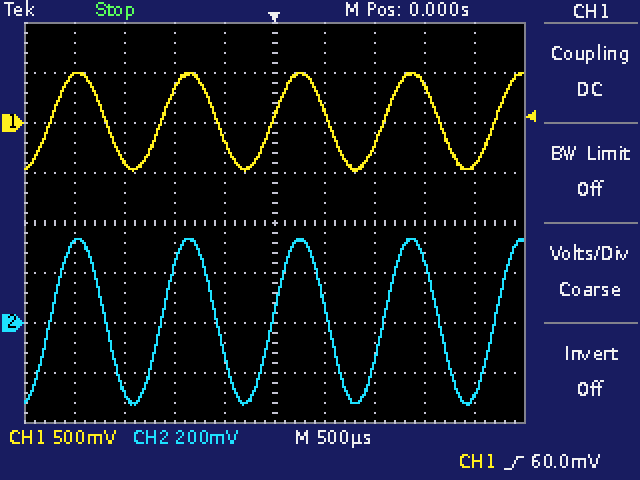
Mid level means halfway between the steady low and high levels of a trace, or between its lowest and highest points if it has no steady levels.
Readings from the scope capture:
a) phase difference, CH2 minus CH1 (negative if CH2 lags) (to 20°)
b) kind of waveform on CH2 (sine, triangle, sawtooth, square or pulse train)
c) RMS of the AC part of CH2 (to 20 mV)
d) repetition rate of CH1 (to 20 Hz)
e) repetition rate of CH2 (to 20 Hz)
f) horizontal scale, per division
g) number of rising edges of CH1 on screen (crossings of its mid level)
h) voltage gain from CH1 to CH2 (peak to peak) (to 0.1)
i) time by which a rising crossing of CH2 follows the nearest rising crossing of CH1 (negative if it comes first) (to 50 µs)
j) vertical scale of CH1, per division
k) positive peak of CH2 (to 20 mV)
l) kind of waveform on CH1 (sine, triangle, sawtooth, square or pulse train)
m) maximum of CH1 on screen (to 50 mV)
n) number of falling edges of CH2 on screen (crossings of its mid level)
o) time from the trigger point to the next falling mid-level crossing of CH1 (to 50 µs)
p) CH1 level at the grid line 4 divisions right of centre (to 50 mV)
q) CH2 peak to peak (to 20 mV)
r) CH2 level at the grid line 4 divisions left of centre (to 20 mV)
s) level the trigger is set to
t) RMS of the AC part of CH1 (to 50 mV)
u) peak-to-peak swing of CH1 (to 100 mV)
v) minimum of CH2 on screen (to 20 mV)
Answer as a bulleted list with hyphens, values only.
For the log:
- 0°
- sine
- 240 mV
- 900 Hz
- 900 Hz
- 500 µs
- 5
- 0.7
- 0 µs
- 500 mV
- 340 mV
- sine
- 500 mV
- 4
- 550 µs
- -400 mV
- 660 mV
- 320 mV
- 60.0 mV
- 350 mV
- 1.00 V
- -320 mV
